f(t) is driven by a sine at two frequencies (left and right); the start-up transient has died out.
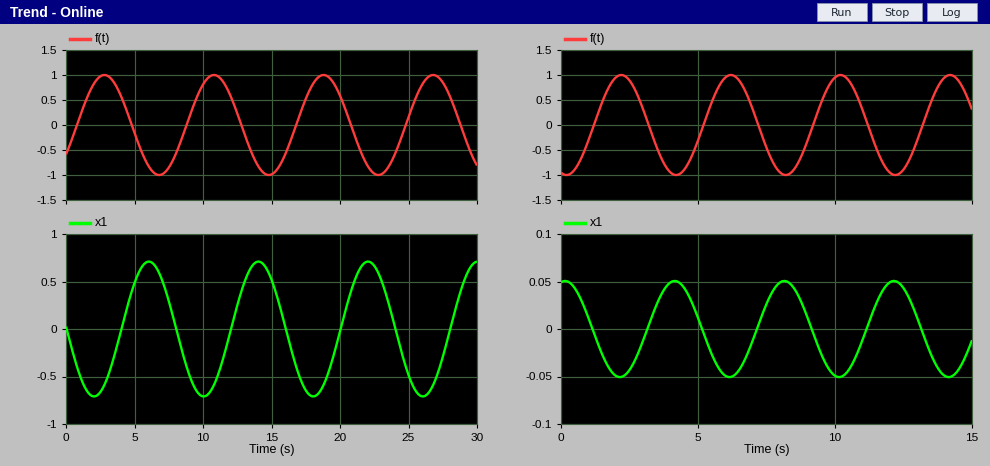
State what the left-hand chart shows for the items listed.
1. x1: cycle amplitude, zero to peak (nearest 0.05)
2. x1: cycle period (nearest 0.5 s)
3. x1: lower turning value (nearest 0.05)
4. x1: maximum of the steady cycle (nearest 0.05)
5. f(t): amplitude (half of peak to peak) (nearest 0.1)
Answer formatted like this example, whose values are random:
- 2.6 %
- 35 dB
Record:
- 0.70
- 8.0 s
- -0.70
- 0.70
- 1.0
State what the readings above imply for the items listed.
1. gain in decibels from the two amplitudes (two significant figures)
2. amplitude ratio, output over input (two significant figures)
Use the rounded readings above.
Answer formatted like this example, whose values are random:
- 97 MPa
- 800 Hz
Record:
- -3.1 dB
- 0.70
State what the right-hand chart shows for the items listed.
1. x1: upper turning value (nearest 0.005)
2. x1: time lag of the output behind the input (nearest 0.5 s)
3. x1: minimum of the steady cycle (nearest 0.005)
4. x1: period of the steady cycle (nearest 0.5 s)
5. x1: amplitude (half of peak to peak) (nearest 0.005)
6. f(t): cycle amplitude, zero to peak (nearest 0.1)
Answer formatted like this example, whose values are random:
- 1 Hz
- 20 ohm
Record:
- 0.050
- 2.0 s
- -0.050
- 4.0 s
- 0.050
- 1.0
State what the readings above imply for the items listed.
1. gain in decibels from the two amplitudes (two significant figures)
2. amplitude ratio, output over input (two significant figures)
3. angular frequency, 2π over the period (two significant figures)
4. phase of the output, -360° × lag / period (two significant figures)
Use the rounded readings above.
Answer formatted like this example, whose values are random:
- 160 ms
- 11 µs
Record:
- -26 dB
- 0.050
- 1.6 rad/s
- -180°
